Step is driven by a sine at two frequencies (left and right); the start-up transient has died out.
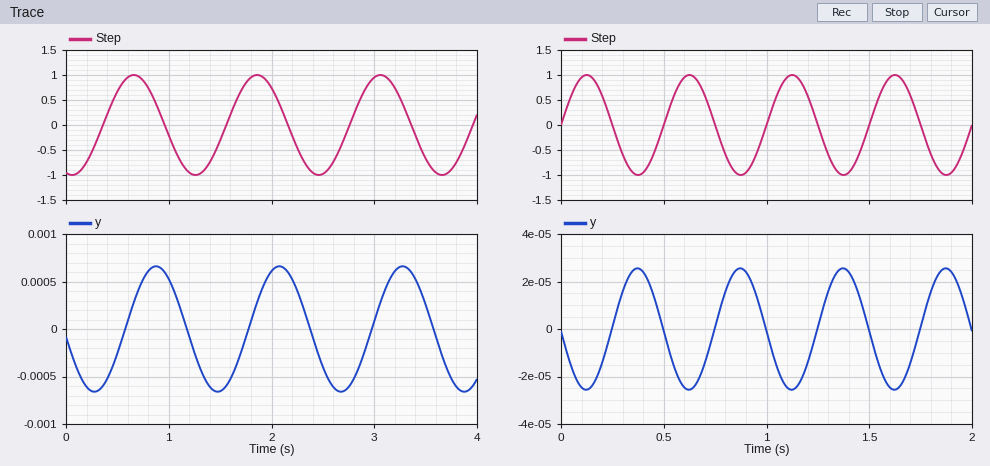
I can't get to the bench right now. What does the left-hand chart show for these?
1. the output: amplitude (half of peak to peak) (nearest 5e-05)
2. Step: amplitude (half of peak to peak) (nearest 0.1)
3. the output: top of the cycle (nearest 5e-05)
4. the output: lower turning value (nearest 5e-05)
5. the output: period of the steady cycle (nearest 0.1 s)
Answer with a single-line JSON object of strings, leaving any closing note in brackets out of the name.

{"the output: amplitude (half of peak to peak)": "0.00065", "Step: amplitude (half of peak to peak)": "1.0", "the output: top of the cycle": "0.00065", "the output: lower turning value": "-0.00065", "the output: period of the steady cycle": "1.2 s"}
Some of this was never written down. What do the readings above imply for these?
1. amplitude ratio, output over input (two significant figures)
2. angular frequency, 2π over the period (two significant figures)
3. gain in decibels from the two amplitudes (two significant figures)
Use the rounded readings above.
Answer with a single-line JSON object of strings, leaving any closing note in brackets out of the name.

{"amplitude ratio, output over input": "0.00065", "angular frequency, 2π over the period": "5.2 rad/s", "gain in decibels from the two amplitudes": "-64 dB"}
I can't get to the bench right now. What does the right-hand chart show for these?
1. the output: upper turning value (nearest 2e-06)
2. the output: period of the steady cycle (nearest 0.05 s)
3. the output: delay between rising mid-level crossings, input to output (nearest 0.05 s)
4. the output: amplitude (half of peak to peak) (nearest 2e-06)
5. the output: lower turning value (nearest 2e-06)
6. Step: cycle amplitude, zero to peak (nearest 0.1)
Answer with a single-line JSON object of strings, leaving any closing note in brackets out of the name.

{"the output: upper turning value": "0.000026", "the output: period of the steady cycle": "0.50 s", "the output: delay between rising mid-level crossings, input to output": "0.25 s", "the output: amplitude (half of peak to peak)": "0.000026", "the output: lower turning value": "-0.000026", "Step: cycle amplitude, zero to peak": "1.0"}
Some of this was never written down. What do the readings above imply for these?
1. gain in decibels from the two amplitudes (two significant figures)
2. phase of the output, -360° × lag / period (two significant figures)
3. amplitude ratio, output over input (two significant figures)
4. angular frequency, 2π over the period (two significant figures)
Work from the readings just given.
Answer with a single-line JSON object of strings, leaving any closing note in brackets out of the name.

{"gain in decibels from the two amplitudes": "-92 dB", "phase of the output, -360° × lag / period": "-180°", "amplitude ratio, output over input": "0.000026", "angular frequency, 2π over the period": "13 rad/s"}
